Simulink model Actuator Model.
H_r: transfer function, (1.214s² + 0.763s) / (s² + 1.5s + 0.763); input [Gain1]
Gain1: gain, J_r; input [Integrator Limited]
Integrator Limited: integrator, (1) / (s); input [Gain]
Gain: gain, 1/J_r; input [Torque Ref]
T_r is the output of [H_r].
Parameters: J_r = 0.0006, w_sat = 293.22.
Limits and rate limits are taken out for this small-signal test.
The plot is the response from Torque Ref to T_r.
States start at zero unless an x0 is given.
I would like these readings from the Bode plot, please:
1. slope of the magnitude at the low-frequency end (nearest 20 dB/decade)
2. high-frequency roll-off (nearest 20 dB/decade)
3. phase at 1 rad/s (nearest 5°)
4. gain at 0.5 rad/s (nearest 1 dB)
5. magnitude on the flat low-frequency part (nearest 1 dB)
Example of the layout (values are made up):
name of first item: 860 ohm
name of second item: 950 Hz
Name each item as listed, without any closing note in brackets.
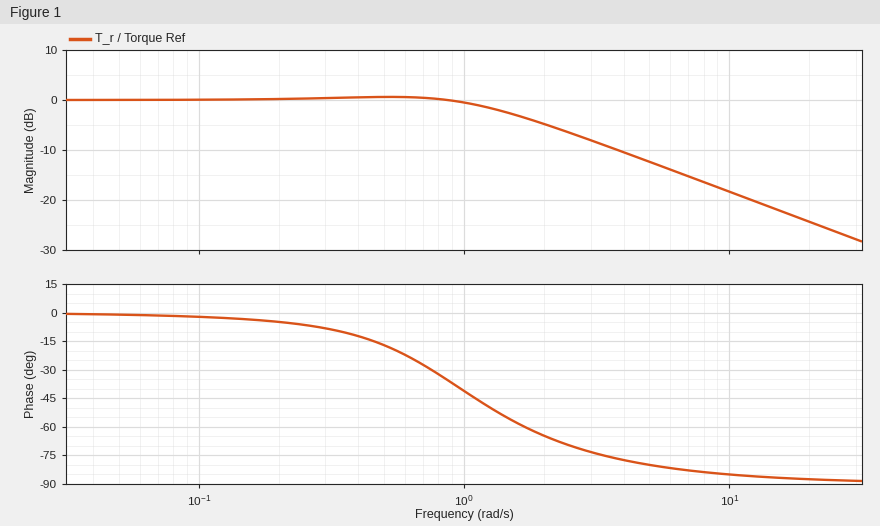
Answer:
slope of the magnitude at the low-frequency end: 0 dB/decade
high-frequency roll-off: -20 dB/decade
phase at 1 rad/s: -40°
gain at 0.5 rad/s: 1 dB
magnitude on the flat low-frequency part: 0 dB
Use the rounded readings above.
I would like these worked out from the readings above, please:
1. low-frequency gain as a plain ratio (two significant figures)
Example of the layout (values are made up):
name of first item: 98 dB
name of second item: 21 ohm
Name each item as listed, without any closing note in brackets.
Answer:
low-frequency gain as a plain ratio: 1.0
